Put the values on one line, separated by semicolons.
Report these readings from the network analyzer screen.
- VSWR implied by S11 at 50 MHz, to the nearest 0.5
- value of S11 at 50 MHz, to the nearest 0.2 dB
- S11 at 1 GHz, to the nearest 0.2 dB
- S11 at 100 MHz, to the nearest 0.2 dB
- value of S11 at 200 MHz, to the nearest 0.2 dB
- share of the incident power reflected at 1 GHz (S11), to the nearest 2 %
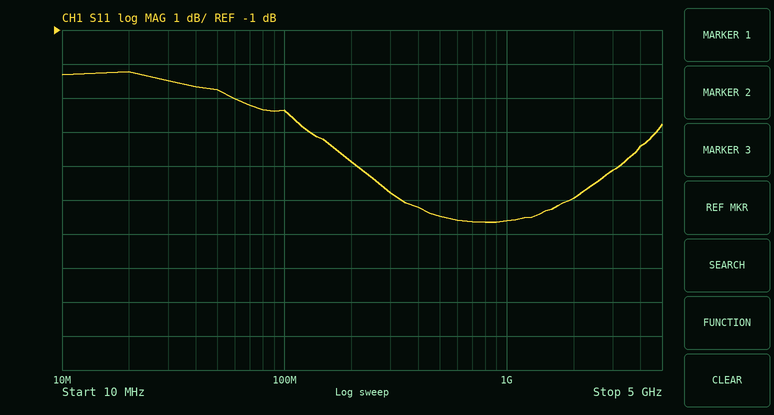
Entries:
6.5; -2.8 dB; -6.6 dB; -3.4 dB; -4.8 dB; 22 %
